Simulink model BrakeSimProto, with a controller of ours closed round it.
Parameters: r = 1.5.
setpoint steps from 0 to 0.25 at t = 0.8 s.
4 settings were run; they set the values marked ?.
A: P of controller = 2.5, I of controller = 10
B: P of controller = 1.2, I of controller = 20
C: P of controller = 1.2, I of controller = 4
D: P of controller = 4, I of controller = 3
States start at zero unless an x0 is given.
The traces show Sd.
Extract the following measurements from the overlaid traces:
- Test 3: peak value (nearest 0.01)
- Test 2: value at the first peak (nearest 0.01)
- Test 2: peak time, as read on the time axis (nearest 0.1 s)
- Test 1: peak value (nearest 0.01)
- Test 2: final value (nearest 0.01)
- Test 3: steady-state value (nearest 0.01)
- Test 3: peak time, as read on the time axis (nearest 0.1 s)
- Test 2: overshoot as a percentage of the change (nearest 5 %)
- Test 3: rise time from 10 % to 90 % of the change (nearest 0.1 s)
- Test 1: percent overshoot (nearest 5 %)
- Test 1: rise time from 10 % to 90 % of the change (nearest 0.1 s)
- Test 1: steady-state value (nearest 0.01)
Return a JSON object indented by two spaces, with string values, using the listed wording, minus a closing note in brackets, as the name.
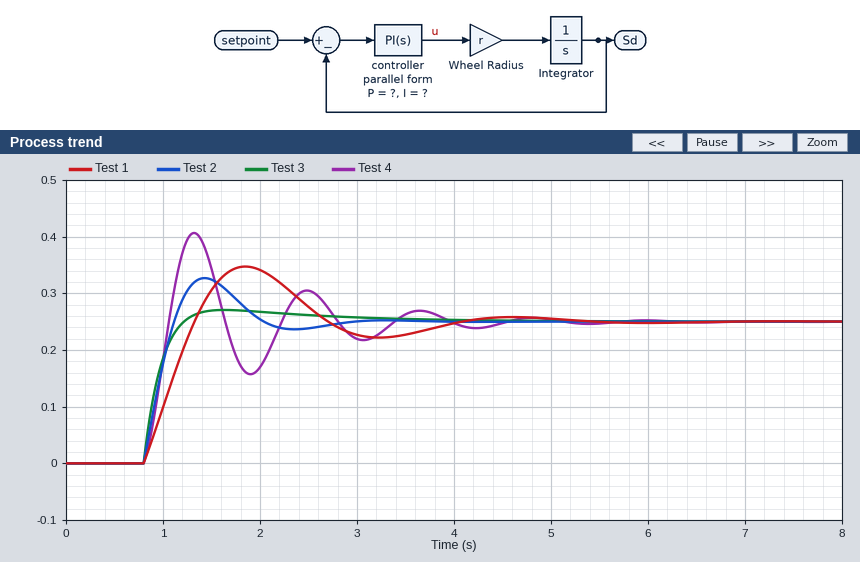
{
  "Test 3: peak value": "0.27",
  "Test 2: value at the first peak": "0.33",
  "Test 2: peak time, as read on the time axis": "1.4 s",
  "Test 1: peak value": "0.35",
  "Test 2: final value": "0.25",
  "Test 3: steady-state value": "0.25",
  "Test 3: peak time, as read on the time axis": "1.6 s",
  "Test 2: overshoot as a percentage of the change": "30 %",
  "Test 3: rise time from 10 % to 90 % of the change": "0.3 s",
  "Test 1: percent overshoot": "40 %",
  "Test 1: rise time from 10 % to 90 % of the change": "0.4 s",
  "Test 1: steady-state value": "0.25"
}
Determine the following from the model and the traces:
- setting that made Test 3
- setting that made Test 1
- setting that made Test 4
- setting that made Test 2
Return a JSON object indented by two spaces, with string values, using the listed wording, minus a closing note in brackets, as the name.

{
  "setting that made Test 3": "D",
  "setting that made Test 1": "C",
  "setting that made Test 4": "B",
  "setting that made Test 2": "A"
}
